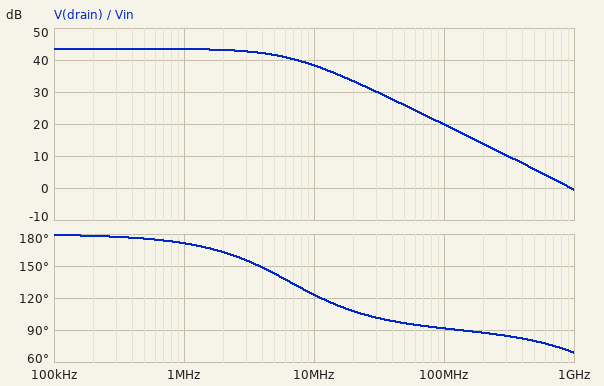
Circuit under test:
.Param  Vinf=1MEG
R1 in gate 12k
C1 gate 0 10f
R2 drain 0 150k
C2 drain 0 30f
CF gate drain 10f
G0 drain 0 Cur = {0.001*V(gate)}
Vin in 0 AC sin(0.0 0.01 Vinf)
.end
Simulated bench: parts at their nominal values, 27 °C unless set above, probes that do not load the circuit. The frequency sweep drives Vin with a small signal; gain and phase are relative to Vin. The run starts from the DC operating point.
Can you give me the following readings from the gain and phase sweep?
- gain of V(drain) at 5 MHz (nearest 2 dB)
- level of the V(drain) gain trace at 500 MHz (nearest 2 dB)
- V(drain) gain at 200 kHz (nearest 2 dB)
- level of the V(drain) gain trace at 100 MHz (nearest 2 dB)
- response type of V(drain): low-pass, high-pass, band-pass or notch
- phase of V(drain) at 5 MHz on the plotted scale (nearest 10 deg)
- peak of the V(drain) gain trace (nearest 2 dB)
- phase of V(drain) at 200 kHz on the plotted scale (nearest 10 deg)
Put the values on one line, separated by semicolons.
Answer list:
42 dB; 6 dB; 44 dB; 20 dB; low-pass; 140 deg; 44 dB; 180 deg
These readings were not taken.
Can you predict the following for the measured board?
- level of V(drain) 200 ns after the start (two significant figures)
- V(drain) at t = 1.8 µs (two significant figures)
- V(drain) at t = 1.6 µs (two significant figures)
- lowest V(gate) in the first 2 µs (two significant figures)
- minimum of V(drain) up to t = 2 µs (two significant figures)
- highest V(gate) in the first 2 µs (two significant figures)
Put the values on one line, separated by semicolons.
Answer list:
-1.3 V; 1.5 V; 680 mV; -9.9 mV; -1.5 V; 9.9 mV
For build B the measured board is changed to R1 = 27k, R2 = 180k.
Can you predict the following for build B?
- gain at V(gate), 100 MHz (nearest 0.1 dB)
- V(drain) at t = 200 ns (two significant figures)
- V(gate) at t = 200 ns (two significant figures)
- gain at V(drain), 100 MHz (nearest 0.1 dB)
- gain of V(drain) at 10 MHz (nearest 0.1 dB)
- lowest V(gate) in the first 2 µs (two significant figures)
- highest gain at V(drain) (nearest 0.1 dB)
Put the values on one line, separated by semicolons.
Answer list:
-17.7 dB; -1.4 V; 7.8 mV; 14.1 dB; 33.8 dB; -9.4 mV; 45.1 dB
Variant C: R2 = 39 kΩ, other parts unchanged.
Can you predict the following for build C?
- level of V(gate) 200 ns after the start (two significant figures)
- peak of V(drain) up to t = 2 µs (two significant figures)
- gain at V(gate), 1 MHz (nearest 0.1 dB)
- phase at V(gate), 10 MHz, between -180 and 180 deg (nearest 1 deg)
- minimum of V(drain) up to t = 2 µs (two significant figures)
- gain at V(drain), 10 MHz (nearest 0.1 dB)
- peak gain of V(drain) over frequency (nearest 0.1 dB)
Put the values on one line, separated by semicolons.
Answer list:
9.4 mV; 390 mV; 0 dB; -17 deg; -390 mV; 31.2 dB; 31.8 dB
